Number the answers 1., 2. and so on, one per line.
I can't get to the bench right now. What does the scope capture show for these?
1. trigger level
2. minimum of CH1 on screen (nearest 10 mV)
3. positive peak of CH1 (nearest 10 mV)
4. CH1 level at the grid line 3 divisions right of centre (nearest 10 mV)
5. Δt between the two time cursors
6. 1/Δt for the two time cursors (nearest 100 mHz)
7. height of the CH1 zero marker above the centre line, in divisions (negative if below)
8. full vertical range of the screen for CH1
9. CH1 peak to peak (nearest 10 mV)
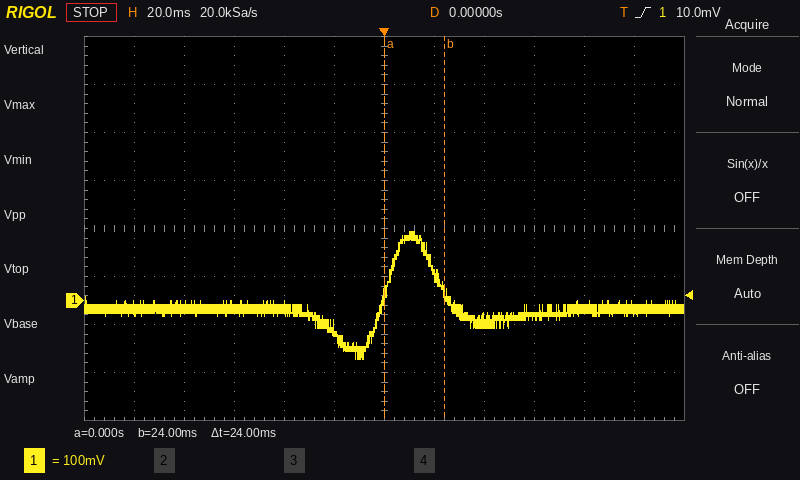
1. 10.0 mV
2. -120 mV
3. 140 mV
4. -30 mV
5. 24 ms
6. 41.7 Hz
7. -1.5 div
8. 800 mV
9. 260 mV
